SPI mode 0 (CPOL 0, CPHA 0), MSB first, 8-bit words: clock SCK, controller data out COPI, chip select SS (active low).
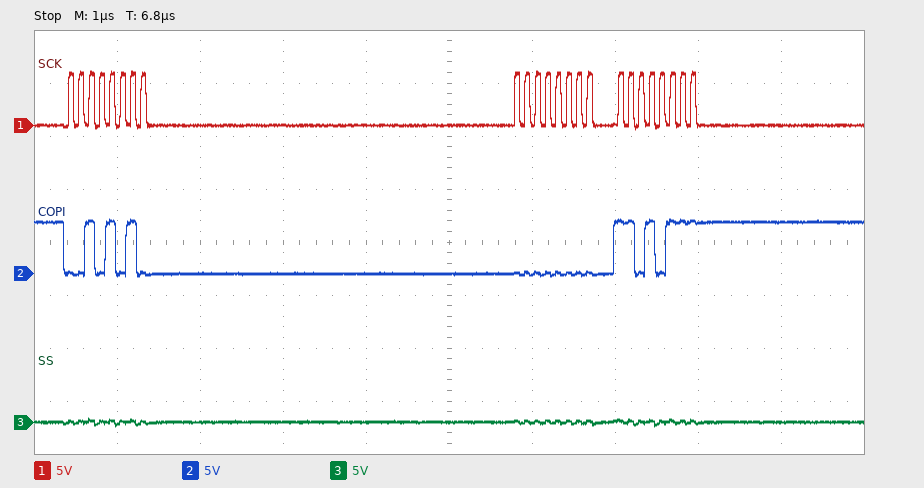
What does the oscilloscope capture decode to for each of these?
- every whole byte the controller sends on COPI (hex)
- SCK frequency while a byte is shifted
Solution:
2A 00 D7
8 MHz
